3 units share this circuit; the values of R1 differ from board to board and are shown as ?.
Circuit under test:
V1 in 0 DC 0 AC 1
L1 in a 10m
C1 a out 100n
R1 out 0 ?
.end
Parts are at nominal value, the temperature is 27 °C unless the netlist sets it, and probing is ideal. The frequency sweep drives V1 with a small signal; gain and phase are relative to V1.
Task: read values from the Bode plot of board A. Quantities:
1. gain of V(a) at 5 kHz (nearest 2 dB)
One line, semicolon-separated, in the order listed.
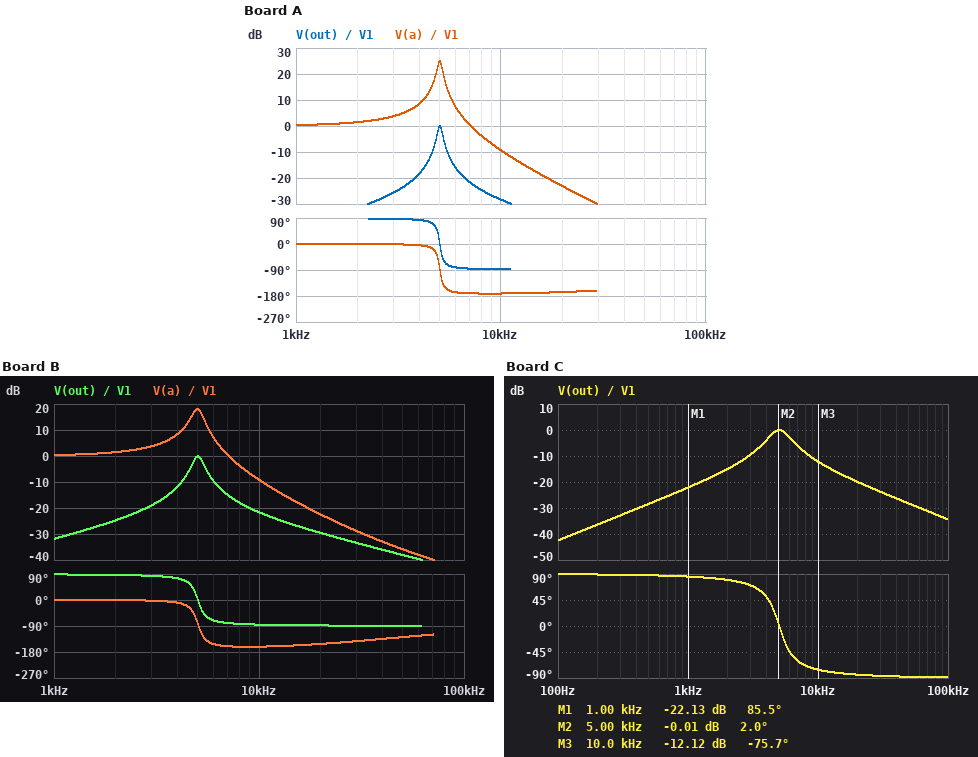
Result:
24 dB
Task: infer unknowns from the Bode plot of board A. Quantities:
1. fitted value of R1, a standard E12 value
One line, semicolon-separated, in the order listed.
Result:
18 Ω
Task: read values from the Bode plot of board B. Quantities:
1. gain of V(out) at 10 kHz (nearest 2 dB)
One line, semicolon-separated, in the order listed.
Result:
-22 dB
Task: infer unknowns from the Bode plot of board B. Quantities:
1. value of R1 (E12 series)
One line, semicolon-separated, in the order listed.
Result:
39 Ω
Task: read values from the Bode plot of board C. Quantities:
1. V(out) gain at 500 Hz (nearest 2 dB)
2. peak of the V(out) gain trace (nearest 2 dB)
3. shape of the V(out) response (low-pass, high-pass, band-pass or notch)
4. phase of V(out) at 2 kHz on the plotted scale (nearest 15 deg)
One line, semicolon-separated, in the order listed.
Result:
-28 dB; 0 dB; band-pass; 75 deg
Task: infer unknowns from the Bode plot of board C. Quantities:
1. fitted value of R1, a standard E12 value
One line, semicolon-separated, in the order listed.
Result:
120 Ω
